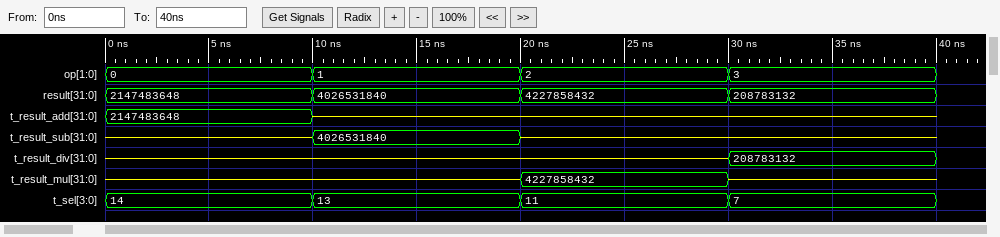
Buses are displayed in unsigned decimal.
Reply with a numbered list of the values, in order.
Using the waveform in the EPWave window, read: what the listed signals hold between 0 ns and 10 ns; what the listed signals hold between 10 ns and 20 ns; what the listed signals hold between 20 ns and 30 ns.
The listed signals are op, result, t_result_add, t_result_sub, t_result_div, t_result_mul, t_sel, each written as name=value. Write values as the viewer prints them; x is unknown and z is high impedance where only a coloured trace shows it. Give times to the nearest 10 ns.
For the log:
1. op=0, result=2147483648, t_result_add=2147483648, t_result_sub=z, t_result_div=z, t_result_mul=z, t_sel=14
2. op=1, result=4026531840, t_result_add=z, t_result_sub=4026531840, t_result_div=z, t_result_mul=z, t_sel=13
3. op=2, result=4227858432, t_result_add=z, t_result_sub=z, t_result_div=z, t_result_mul=4227858432, t_sel=11
